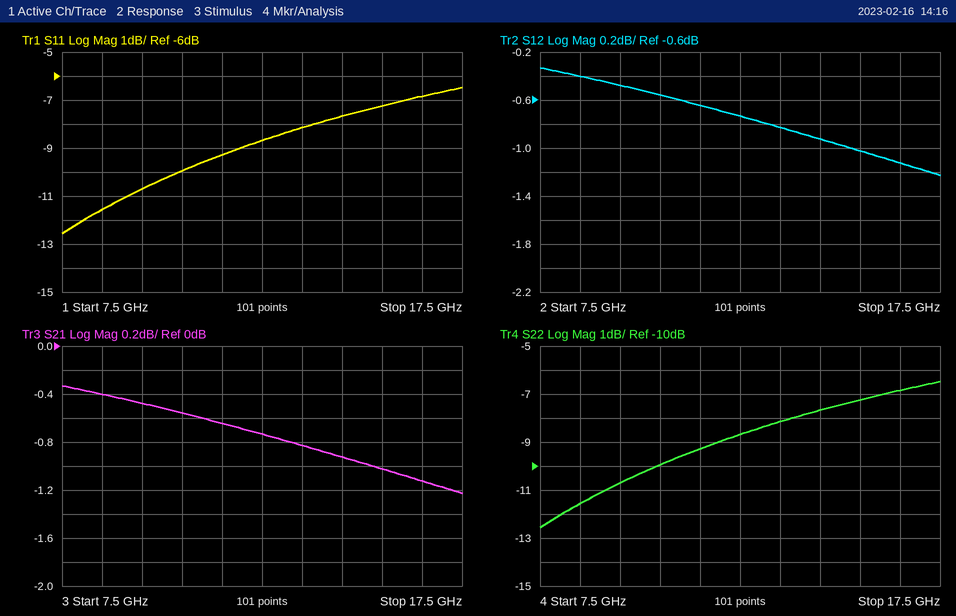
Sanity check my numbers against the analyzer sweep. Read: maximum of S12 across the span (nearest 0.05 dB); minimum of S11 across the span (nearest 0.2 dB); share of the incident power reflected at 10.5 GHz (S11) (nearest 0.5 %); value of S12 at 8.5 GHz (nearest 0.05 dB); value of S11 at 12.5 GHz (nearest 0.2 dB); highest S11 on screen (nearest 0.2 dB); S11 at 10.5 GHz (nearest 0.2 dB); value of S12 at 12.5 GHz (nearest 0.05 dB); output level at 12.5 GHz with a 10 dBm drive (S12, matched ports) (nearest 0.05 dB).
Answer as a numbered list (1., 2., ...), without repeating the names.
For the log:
1. -0.35 dB
2. -12.6 dB
3. 10.0 %
4. -0.40 dB
5. -8.6 dB
6. -6.4 dB
7. -10.0 dB
8. -0.75 dB
9. 9.25 dBm
